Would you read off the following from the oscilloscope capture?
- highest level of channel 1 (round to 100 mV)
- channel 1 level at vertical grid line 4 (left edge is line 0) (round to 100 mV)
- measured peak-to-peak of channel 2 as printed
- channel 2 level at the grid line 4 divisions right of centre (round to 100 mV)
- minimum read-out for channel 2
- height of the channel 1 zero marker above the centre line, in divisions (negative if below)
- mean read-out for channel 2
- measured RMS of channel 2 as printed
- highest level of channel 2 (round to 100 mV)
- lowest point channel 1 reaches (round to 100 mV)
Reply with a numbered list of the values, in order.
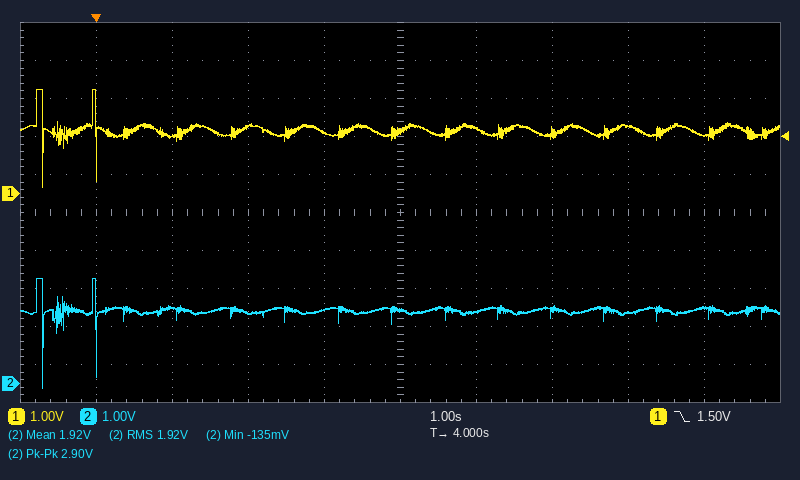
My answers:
1. 2.7 V
2. 1.6 V
3. 2.90 V
4. 2.0 V
5. -135 mV
6. +0.5 div
7. 1.92 V
8. 1.92 V
9. 2.8 V
10. 200 mV
